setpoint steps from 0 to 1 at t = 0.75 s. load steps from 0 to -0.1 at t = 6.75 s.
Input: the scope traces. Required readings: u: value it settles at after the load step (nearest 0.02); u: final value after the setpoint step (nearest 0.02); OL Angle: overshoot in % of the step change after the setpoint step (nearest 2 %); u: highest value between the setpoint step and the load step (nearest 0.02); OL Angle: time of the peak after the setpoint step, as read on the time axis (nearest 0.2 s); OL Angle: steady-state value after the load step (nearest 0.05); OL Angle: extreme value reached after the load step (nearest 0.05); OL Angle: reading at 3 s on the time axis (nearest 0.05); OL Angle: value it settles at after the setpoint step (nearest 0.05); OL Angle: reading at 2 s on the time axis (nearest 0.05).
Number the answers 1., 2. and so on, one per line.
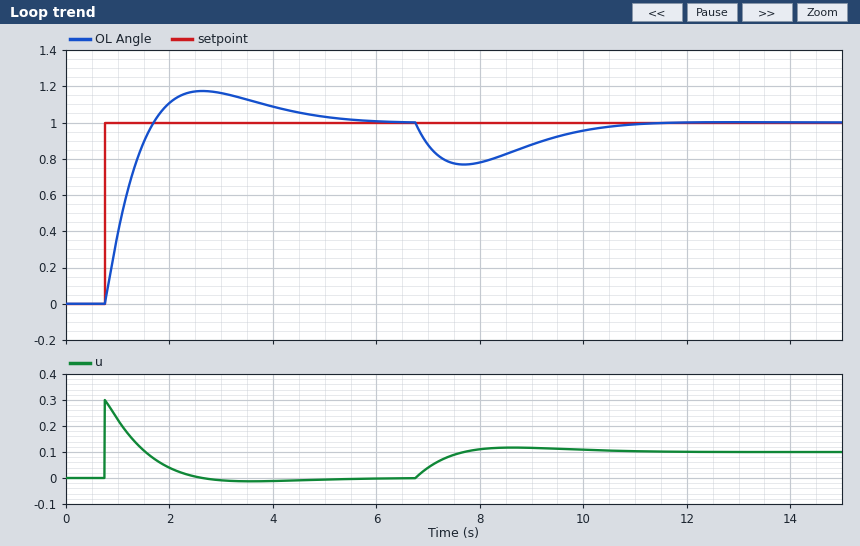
1. 0.10
2. 0.00
3. 18 %
4. 0.30
5. 2.6 s
6. 1.00
7. 0.75
8. 1.15
9. 1.00
10. 1.10
